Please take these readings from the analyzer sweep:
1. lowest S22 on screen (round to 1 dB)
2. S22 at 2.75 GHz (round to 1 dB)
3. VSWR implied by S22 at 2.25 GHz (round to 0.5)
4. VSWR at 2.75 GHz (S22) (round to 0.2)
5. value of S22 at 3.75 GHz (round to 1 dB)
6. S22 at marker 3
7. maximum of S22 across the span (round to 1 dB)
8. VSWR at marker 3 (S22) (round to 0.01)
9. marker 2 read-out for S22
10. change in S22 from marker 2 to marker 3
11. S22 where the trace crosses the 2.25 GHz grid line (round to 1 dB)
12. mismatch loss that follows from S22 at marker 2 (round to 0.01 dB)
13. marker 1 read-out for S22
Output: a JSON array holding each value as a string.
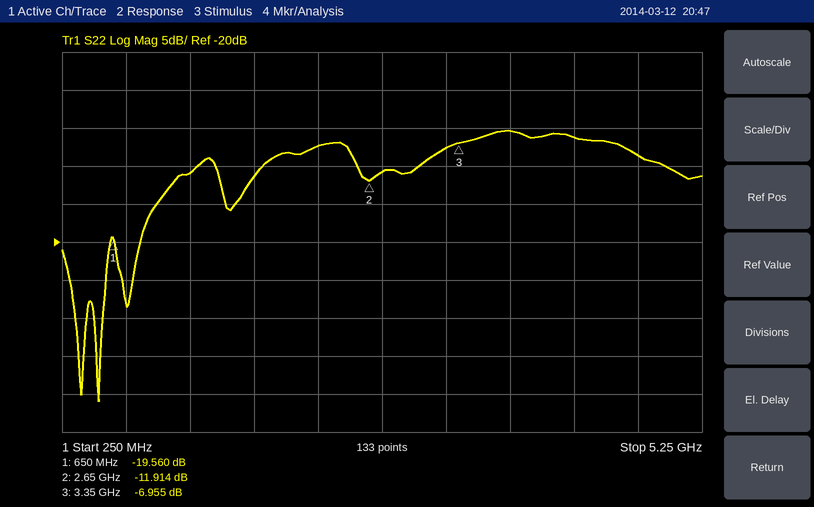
["-41 dB", "-11 dB", "2.5", "1.8", "-5 dB", "-6.955 dB", "-5 dB", "2.63", "-11.914 dB", "4.959 dB", "-7 dB", "0.29 dB", "-19.560 dB"]
